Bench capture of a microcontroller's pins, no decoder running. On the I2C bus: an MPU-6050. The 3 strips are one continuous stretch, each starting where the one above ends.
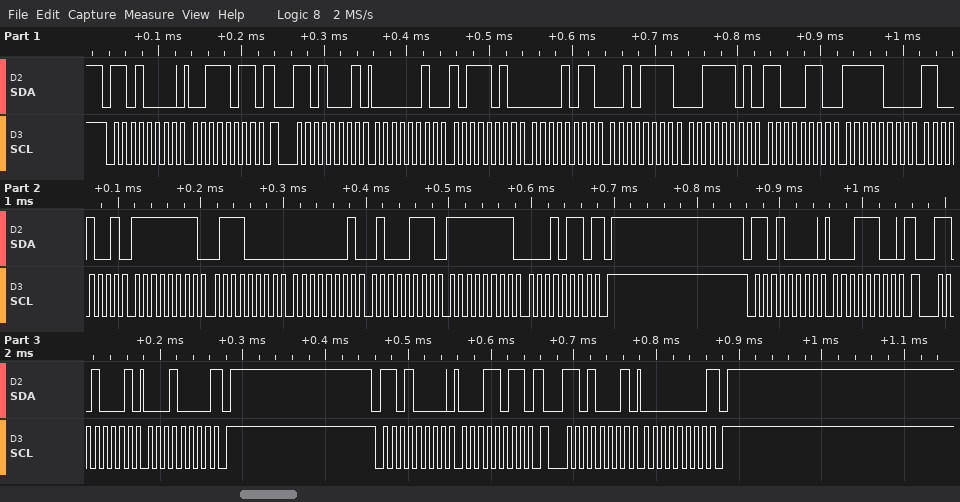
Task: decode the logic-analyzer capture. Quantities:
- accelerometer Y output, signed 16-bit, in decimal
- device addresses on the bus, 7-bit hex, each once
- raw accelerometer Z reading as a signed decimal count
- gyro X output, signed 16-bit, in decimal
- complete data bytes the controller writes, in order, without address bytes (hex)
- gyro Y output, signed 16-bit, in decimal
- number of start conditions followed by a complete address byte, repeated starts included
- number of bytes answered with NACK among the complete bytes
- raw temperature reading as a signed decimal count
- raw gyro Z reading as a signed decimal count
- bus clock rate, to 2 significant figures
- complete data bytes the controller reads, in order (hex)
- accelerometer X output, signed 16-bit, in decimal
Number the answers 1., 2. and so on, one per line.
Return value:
1. 2863
2. 0x68
3. 15814
4. -144
5. 3B 1C 1B
6. 327
7. 6
8. 3
9. -1847
10. -234
11. 100 kHz
12. 02 BA 0B 2F 3D C6 F8 C9 FF 70 01 47 FF 16 10 00
13. 698
